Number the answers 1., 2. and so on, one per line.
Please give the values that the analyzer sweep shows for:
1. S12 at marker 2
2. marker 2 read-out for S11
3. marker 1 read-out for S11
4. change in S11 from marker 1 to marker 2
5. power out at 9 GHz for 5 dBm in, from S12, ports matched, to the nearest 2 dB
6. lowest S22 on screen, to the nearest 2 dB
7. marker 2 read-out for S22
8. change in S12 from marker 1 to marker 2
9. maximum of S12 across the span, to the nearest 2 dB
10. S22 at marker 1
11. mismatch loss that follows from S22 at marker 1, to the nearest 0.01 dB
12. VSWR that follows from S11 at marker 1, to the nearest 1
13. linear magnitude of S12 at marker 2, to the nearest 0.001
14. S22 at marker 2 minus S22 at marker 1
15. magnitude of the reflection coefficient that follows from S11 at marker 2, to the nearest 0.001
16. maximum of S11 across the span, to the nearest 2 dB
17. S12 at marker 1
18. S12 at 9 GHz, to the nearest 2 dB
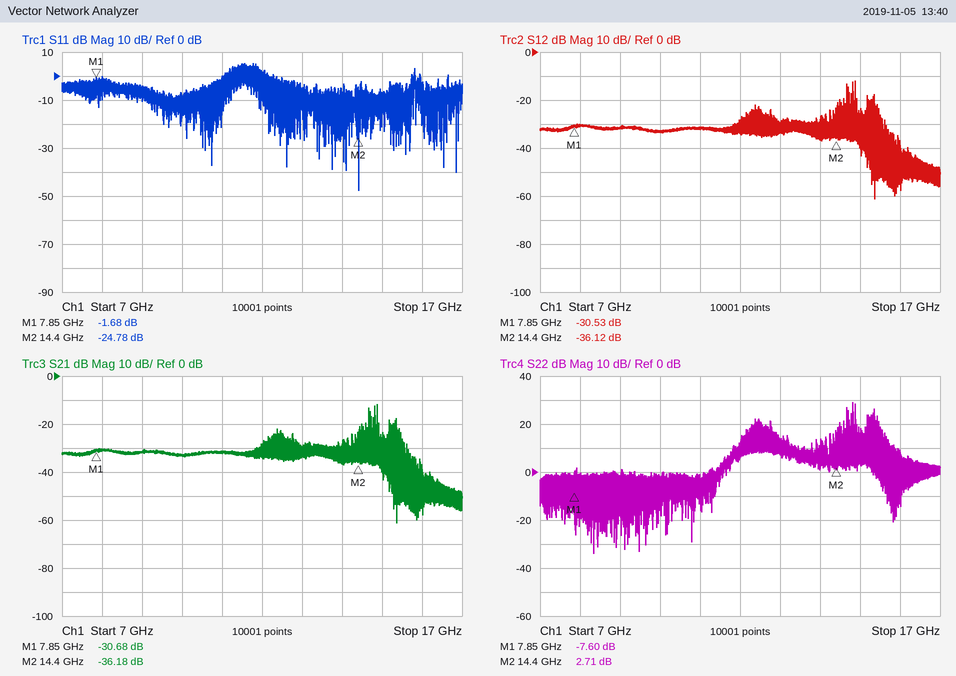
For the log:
1. -36.12 dB
2. -24.78 dB
3. -1.68 dB
4. -23.10 dB
5. -26 dBm
6. -34 dB
7. 2.71 dB
8. -5.59 dB
9. -12 dB
10. -7.60 dB
11. 0.83 dB
12. 10
13. 0.016
14. 10.31 dB
15. 0.058
16. 6 dB
17. -30.53 dB
18. -32 dB
